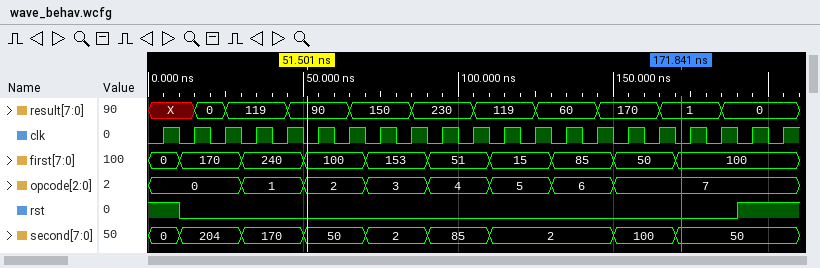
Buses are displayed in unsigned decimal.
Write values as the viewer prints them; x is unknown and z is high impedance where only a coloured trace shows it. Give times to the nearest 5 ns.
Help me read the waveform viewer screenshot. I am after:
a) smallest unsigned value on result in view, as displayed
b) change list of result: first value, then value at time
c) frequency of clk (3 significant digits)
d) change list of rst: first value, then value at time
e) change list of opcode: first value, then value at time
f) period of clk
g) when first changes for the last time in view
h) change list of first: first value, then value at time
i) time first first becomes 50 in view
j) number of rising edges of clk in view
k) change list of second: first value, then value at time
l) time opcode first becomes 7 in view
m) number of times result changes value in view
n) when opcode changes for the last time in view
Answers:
0
X, 0 at 15 ns, 119 at 25 ns, 90 at 45 ns, 150 at 65 ns, 230 at 85 ns, 119 at 105 ns, 60 at 125 ns, 170 at 145 ns, 1 at 165 ns, 0 at 185 ns
100 MHz
1, 0 at 10 ns, 1 at 190 ns
0, 1 at 30 ns, 2 at 50 ns, 3 at 70 ns, 4 at 90 ns, 5 at 110 ns, 6 at 130 ns, 7 at 150 ns
10 ns
170 ns
0, 170 at 10 ns, 240 at 30 ns, 100 at 50 ns, 153 at 70 ns, 51 at 90 ns, 15 at 110 ns, 85 at 130 ns, 50 at 150 ns, 100 at 170 ns
150 ns
21
0, 204 at 10 ns, 170 at 30 ns, 50 at 50 ns, 2 at 70 ns, 85 at 90 ns, 2 at 110 ns, 100 at 150 ns, 50 at 170 ns
150 ns
10
150 ns
